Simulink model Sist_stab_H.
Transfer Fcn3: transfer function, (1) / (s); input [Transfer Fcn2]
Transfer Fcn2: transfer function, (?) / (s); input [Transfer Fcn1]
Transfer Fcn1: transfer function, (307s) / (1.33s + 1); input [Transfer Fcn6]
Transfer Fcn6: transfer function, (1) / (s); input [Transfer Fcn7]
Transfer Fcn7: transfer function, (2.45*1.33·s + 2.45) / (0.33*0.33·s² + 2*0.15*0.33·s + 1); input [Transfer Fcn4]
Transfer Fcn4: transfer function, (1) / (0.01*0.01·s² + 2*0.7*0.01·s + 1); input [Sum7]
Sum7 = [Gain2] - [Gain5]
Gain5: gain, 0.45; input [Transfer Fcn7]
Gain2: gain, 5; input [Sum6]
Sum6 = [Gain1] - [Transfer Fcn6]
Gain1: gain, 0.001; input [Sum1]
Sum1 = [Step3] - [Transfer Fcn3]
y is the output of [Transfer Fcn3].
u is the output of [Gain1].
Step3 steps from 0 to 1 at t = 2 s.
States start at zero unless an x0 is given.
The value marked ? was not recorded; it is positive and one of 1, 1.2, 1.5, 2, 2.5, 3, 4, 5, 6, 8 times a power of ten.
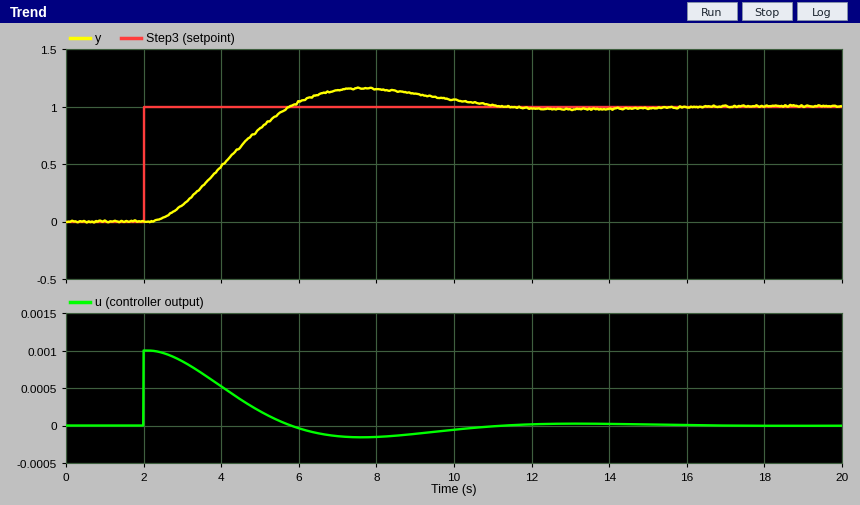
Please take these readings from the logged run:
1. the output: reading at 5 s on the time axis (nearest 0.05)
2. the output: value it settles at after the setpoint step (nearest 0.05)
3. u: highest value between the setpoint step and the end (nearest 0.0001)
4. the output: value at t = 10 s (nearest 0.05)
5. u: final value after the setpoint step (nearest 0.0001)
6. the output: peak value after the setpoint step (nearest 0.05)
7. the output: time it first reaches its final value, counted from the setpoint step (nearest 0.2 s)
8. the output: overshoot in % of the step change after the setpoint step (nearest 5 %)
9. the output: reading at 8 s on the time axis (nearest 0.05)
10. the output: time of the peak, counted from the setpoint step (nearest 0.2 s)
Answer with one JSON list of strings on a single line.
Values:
["0.80", "1.00", "0.0010", "1.05", "0.0000", "1.15", "3.8 s", "15 %", "1.15", "5.6 s"]
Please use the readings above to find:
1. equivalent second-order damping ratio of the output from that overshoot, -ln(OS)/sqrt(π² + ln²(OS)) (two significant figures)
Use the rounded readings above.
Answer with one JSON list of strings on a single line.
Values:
["0.52"]
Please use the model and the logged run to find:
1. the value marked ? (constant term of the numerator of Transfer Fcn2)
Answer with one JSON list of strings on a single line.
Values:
["2"]
